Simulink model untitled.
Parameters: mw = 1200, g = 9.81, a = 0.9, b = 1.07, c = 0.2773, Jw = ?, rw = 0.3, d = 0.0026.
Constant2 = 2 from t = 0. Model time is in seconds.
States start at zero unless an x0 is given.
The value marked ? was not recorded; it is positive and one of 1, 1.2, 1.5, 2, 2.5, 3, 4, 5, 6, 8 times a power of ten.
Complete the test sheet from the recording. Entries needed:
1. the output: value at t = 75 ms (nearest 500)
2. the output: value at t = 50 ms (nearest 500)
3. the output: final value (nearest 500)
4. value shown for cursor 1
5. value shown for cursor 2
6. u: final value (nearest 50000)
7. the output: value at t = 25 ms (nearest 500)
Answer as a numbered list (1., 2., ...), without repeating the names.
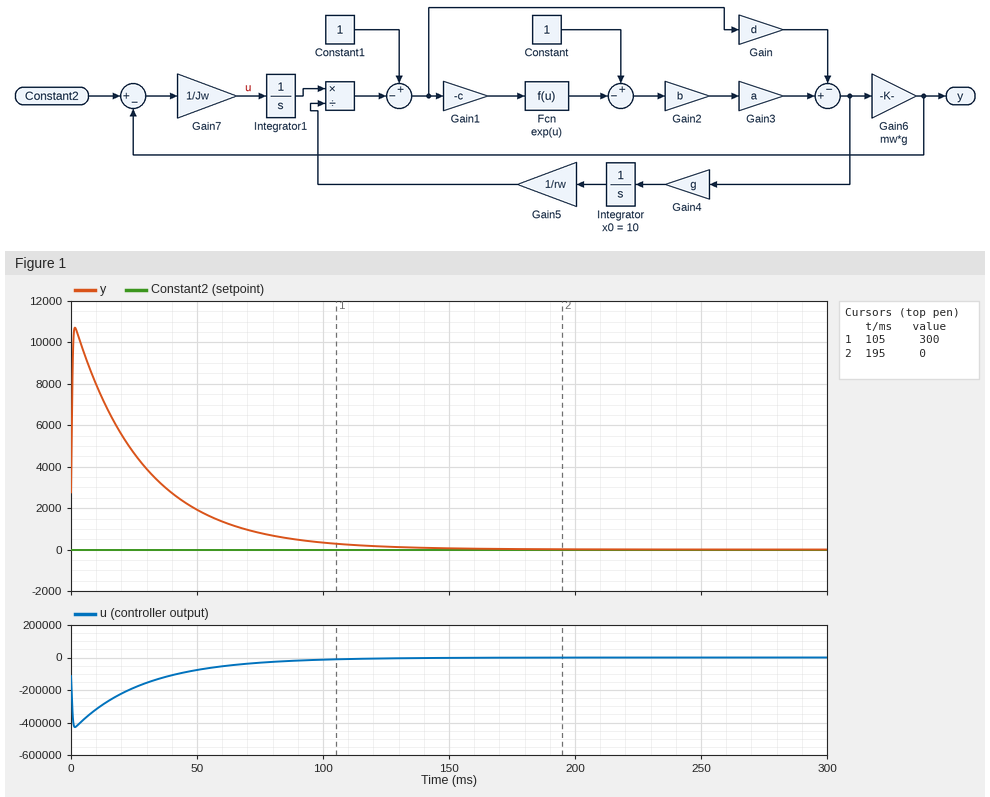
1. 1000
2. 2000
3. 0
4. 300
5. 0
6. 0
7. 4500
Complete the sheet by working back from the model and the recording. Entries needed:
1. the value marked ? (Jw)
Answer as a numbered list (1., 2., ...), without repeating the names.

1. 0.025
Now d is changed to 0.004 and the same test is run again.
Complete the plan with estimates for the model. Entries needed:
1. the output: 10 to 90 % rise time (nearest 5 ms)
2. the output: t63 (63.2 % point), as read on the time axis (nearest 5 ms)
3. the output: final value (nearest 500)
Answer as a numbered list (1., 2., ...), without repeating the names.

1. 40 ms
2. 45 ms
3. 0
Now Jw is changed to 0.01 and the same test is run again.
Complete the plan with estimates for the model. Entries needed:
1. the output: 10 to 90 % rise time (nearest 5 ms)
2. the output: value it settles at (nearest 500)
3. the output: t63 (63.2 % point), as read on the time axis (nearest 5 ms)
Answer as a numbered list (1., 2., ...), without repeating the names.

1. 25 ms
2. 0
3. 25 ms
